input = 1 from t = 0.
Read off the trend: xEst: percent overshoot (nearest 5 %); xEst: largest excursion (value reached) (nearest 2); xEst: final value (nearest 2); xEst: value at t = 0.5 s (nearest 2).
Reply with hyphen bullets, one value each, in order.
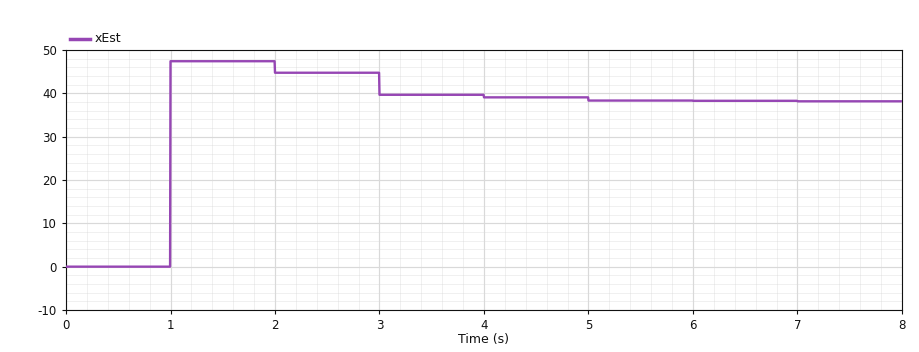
- 25 %
- 48
- 38
- 0
